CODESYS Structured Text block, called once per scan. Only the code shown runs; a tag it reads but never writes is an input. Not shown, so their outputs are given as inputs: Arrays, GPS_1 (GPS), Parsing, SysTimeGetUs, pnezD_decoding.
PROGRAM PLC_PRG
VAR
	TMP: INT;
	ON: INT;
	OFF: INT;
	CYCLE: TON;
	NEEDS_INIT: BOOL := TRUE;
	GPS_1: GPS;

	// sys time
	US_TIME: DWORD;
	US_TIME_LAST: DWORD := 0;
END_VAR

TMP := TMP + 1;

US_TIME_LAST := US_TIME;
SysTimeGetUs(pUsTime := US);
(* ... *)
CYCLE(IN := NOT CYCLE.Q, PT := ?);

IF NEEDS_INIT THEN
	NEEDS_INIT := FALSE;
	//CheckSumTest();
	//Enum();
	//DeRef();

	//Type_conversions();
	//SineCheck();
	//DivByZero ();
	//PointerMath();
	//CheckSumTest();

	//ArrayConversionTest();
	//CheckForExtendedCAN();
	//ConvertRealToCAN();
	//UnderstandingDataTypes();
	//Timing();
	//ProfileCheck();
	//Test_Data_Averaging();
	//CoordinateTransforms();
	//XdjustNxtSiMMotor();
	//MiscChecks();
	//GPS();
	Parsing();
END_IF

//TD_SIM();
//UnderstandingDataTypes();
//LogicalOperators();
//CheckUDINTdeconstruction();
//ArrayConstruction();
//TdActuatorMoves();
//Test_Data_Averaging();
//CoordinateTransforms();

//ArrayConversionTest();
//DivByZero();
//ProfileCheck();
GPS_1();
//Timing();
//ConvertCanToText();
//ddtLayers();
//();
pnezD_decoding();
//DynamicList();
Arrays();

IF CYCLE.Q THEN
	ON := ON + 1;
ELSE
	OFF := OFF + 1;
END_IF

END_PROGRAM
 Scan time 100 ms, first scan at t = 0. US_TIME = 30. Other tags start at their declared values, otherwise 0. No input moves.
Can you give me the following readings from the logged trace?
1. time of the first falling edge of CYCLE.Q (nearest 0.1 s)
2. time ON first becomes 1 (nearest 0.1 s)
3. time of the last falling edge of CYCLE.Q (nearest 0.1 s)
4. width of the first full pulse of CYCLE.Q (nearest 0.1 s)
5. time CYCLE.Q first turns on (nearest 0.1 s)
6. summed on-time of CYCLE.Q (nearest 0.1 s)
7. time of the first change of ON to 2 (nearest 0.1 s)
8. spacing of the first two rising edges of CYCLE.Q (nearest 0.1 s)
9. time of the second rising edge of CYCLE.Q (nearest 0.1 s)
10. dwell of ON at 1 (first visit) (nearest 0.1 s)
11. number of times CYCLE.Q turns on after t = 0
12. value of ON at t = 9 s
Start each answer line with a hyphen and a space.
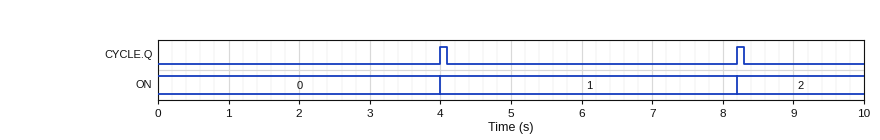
- 4.1 s
- 4.0 s
- 8.3 s
- 0.1 s
- 4.0 s
- 0.2 s
- 8.2 s
- 4.2 s
- 8.2 s
- 4.2 s
- 2
- 2
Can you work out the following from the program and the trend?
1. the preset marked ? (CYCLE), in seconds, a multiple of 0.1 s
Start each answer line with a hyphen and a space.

- 4.0 s
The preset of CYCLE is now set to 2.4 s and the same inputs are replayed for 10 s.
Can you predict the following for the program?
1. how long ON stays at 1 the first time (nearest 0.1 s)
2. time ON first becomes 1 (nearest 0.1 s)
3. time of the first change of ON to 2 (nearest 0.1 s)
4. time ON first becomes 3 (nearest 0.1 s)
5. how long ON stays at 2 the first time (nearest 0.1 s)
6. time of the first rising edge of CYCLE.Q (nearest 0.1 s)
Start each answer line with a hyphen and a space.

- 2.6 s
- 2.4 s
- 5.0 s
- 7.6 s
- 2.6 s
- 2.4 s
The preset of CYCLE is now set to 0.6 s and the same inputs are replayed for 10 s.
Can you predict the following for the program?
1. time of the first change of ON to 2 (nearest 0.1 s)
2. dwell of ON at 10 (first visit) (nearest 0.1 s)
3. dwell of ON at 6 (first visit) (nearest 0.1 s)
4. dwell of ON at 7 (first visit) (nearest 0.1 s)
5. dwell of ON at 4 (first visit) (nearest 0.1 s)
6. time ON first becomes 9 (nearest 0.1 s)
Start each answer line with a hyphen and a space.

- 1.4 s
- 0.8 s
- 0.8 s
- 0.8 s
- 0.8 s
- 7.0 s
